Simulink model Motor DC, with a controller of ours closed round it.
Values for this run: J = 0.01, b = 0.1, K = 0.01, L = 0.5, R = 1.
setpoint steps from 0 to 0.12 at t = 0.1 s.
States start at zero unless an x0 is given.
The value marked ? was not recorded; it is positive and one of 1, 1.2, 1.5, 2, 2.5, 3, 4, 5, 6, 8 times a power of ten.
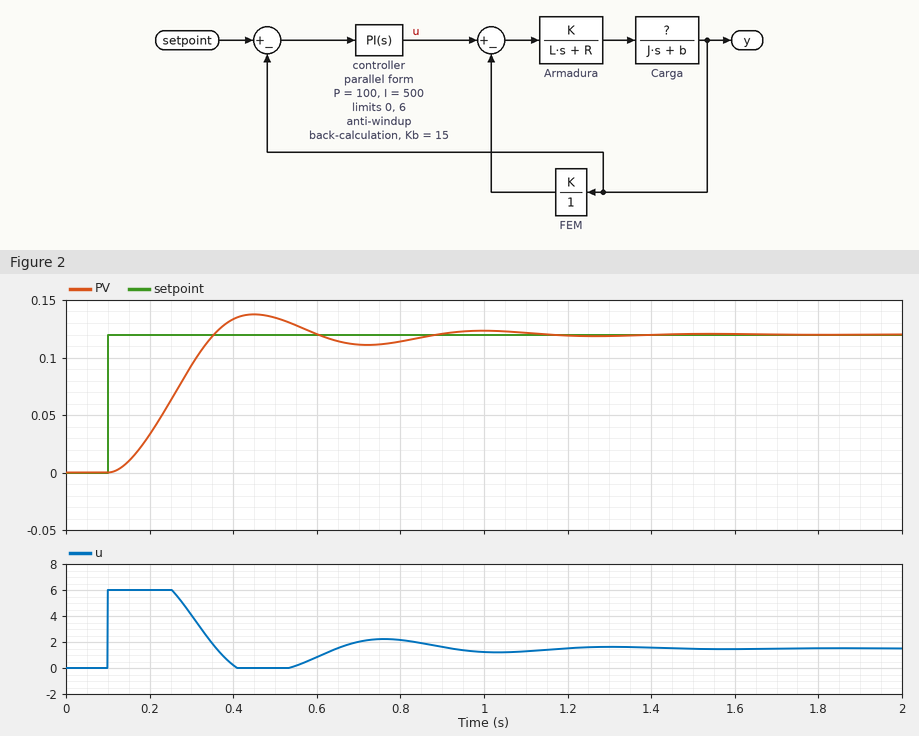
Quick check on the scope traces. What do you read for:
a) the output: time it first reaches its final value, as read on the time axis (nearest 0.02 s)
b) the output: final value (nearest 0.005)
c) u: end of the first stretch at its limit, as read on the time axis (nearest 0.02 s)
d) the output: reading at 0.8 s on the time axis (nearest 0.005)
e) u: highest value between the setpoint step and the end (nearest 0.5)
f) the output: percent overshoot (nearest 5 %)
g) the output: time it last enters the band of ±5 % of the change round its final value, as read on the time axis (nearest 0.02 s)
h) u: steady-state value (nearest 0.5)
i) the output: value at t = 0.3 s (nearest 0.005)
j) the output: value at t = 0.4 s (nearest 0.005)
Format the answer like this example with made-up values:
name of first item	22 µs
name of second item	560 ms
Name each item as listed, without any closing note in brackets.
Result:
the output: time it first reaches its final value, as read on the time axis	0.36 s
the output: final value	0.120
u: end of the first stretch at its limit, as read on the time axis	0.26 s
the output: reading at 0.8 s on the time axis	0.115
u: highest value between the setpoint step and the end	6.0
the output: percent overshoot	15 %
the output: time it last enters the band of ±5 % of the change round its final value, as read on the time axis	0.80 s
u: steady-state value	1.5
the output: value at t = 0.3 s	0.095
the output: value at t = 0.4 s	0.135
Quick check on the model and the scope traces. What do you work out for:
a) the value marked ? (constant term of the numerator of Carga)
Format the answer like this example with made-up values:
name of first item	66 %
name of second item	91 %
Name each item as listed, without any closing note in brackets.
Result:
the value marked ?	0.8
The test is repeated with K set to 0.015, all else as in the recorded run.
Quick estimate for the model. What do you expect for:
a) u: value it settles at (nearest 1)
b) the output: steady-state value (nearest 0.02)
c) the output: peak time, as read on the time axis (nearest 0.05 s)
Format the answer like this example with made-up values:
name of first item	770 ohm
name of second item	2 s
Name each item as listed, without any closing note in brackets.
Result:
u: value it settles at	1
the output: steady-state value	0.12
the output: peak time, as read on the time axis	0.40 s
